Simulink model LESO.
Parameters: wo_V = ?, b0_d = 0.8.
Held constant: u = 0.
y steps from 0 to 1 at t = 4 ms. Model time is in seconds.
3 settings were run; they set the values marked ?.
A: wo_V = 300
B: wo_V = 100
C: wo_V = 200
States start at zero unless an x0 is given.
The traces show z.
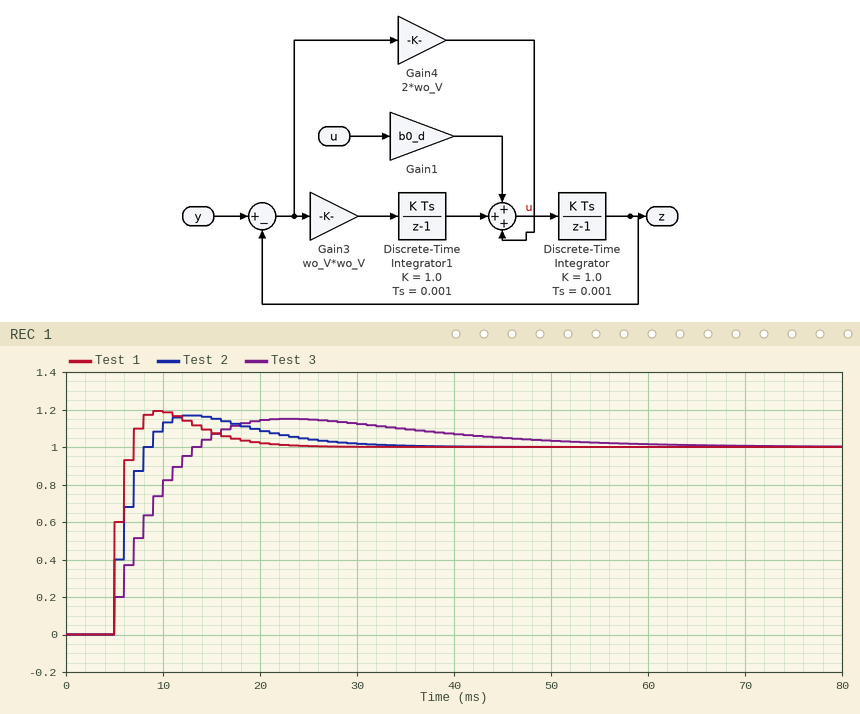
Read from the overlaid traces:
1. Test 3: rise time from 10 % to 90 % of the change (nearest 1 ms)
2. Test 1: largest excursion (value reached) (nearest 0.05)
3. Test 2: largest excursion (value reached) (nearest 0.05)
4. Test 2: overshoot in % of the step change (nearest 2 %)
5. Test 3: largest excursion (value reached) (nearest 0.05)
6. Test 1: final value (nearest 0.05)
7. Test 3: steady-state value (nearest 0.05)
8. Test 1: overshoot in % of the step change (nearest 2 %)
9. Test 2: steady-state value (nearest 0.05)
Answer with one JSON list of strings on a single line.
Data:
["7 ms", "1.20", "1.15", "16 %", "1.15", "1.00", "1.00", "20 %", "1.00"]
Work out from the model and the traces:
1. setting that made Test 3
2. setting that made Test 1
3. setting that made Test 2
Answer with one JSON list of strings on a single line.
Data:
["B", "A", "C"]
